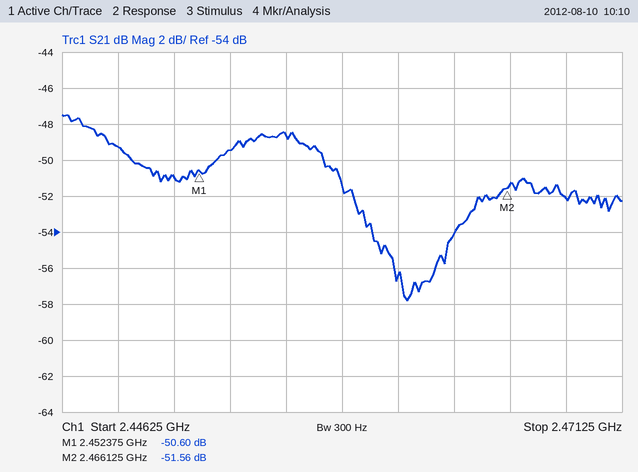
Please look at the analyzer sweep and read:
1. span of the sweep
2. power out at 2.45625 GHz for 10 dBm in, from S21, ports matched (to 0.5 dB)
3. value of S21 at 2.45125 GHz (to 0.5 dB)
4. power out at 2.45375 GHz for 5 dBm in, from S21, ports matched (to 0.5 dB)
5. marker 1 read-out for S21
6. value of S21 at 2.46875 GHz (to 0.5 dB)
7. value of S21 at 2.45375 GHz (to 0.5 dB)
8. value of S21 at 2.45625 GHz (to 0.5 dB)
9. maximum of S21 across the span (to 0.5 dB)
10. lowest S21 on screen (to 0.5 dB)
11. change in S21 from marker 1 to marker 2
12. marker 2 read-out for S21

25 MHz
-38.5 dBm
-51.0 dB
-44.5 dBm
-50.60 dB
-52.0 dB
-49.5 dB
-48.5 dB
-47.5 dB
-58.0 dB
-0.96 dB
-51.56 dB
